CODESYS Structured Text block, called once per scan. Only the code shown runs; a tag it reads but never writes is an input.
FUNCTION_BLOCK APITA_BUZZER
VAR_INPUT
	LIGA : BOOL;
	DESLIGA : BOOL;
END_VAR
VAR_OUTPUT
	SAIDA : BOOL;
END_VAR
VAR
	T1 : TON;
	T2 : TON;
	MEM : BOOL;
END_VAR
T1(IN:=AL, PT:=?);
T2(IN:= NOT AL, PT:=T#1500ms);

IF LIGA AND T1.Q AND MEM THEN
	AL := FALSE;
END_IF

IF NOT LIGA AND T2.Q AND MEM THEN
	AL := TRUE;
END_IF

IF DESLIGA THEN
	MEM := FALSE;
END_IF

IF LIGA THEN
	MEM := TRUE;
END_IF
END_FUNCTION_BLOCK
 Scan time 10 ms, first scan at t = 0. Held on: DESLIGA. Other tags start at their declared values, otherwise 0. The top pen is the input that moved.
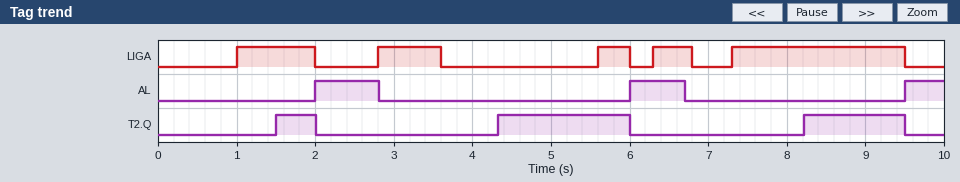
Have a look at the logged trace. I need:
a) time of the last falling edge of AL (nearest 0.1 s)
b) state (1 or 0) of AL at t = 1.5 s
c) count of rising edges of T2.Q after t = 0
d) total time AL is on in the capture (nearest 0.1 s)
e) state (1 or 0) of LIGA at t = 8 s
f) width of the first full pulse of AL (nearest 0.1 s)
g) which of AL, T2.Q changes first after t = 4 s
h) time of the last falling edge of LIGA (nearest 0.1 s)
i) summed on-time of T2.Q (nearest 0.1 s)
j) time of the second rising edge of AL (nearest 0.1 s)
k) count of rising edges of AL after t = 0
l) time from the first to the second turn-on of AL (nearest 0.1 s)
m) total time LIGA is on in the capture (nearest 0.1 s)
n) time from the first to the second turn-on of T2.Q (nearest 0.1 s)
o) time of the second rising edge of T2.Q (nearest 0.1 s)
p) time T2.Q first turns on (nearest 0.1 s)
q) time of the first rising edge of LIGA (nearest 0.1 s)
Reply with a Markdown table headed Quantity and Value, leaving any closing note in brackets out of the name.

| Quantity | Value |
|---|---|
| time of the last falling edge of AL | 6.7 s |
| state (1 or 0) of AL at t = 1.5 s | 0 |
| count of rising edges of T2.Q after t = 0 | 3 |
| total time AL is on in the capture | 2.0 s |
| state (1 or 0) of LIGA at t = 8 s | 1 |
| width of the first full pulse of AL | 0.8 s |
| which of AL, T2.Q changes first after t = 4 s | T2.Q |
| time of the last falling edge of LIGA | 9.5 s |
| summed on-time of T2.Q | 3.5 s |
| time of the second rising edge of AL | 6.0 s |
| count of rising edges of AL after t = 0 | 3 |
| time from the first to the second turn-on of AL | 4.0 s |
| total time LIGA is on in the capture | 4.9 s |
| time from the first to the second turn-on of T2.Q | 2.8 s |
| time of the second rising edge of T2.Q | 4.3 s |
| time T2.Q first turns on | 1.5 s |
| time of the first rising edge of LIGA | 1.0 s |
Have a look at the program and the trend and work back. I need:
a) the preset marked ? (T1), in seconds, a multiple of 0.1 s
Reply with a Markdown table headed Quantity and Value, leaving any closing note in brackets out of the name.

| Quantity | Value |
|---|---|
| the preset marked ? (T1), in seconds, a multiple of 0.1 s | 0.7 s |
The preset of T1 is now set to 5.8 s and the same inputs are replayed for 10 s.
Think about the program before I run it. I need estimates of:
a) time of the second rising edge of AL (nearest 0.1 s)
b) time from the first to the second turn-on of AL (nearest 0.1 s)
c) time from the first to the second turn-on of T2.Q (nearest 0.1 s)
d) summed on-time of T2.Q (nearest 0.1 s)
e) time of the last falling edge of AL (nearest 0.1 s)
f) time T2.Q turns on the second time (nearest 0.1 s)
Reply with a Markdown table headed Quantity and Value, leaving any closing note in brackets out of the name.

| Quantity | Value |
|---|---|
| time of the second rising edge of AL | 9.5 s |
| time from the first to the second turn-on of AL | 7.5 s |
| time from the first to the second turn-on of T2.Q | 7.8 s |
| summed on-time of T2.Q | 0.7 s |
| time of the last falling edge of AL | 7.8 s |
| time T2.Q turns on the second time | 9.3 s |
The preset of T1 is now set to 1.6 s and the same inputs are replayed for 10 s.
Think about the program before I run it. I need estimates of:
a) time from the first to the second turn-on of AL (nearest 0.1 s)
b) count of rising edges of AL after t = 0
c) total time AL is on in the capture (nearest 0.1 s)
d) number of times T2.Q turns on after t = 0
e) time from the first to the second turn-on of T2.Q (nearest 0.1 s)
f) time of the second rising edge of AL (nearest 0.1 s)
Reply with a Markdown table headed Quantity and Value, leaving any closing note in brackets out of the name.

| Quantity | Value |
|---|---|
| time from the first to the second turn-on of AL | 7.5 s |
| count of rising edges of AL after t = 0 | 2 |
| total time AL is on in the capture | 4.1 s |
| number of times T2.Q turns on after t = 0 | 2 |
| time from the first to the second turn-on of T2.Q | 5.6 s |
| time of the second rising edge of AL | 9.5 s |
